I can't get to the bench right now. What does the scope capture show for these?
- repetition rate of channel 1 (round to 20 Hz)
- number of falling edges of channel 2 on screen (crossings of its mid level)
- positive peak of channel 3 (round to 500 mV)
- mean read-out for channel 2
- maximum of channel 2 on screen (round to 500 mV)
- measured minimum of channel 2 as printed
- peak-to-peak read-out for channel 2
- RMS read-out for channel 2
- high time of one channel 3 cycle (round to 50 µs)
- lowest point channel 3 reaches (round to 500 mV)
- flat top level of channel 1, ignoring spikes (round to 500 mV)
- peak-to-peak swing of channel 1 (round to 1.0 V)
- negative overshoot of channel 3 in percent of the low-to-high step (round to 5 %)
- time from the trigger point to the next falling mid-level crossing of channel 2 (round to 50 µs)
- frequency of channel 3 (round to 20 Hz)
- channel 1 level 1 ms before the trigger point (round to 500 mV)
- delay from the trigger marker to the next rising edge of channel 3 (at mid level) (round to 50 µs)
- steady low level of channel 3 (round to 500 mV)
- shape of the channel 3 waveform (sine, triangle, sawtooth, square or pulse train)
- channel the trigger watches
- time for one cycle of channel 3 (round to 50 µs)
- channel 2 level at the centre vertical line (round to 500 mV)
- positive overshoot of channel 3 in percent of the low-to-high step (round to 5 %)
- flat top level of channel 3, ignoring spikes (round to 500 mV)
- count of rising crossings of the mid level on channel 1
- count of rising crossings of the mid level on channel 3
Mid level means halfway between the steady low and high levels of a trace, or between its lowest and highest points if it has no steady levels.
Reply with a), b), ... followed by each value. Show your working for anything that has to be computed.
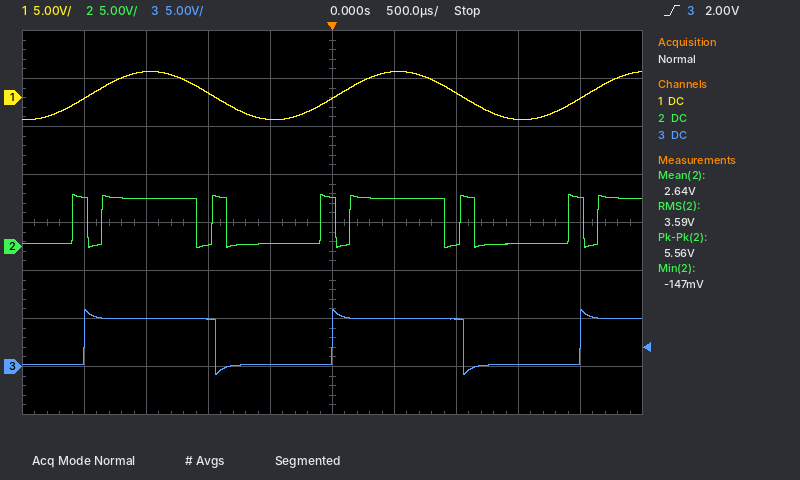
a) 1 / 2.00 ms ≈ 500 Hz
b) 7
c) 6.0 V
d) 2.64 V
e) 5.5 V
f) -147 mV
g) 5.56 V
h) 3.59 V
i) 1.05 ms
j) -1.0 V
k) 2.5 V
l) 5.0 V
m) 20 %
n) 50 µs
o) 1 / 2.00 ms ≈ 500 Hz
p) 500 mV
q) 2.00 ms
r) 0.0 V
s) square
t) channel 3
u) 2.00 ms
v) 5.0 V
w) 20 %
x) 5.0 V
y) 3
z) 3
